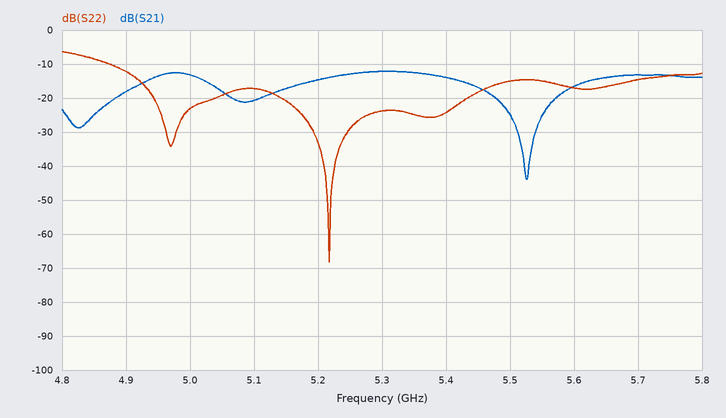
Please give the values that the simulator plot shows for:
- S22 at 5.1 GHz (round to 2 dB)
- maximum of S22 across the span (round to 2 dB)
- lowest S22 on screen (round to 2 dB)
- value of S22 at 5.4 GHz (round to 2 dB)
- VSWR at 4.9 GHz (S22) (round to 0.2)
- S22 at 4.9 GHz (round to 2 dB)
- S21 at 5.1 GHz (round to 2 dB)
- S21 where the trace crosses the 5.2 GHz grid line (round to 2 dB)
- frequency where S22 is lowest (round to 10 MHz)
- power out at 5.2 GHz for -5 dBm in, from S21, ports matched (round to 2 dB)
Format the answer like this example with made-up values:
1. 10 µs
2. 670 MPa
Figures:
1. -18 dB
2. -6 dB
3. -68 dB
4. -24 dB
5. 1.6
6. -12 dB
7. -20 dB
8. -14 dB
9. 5.22 GHz
10. -20 dBm
